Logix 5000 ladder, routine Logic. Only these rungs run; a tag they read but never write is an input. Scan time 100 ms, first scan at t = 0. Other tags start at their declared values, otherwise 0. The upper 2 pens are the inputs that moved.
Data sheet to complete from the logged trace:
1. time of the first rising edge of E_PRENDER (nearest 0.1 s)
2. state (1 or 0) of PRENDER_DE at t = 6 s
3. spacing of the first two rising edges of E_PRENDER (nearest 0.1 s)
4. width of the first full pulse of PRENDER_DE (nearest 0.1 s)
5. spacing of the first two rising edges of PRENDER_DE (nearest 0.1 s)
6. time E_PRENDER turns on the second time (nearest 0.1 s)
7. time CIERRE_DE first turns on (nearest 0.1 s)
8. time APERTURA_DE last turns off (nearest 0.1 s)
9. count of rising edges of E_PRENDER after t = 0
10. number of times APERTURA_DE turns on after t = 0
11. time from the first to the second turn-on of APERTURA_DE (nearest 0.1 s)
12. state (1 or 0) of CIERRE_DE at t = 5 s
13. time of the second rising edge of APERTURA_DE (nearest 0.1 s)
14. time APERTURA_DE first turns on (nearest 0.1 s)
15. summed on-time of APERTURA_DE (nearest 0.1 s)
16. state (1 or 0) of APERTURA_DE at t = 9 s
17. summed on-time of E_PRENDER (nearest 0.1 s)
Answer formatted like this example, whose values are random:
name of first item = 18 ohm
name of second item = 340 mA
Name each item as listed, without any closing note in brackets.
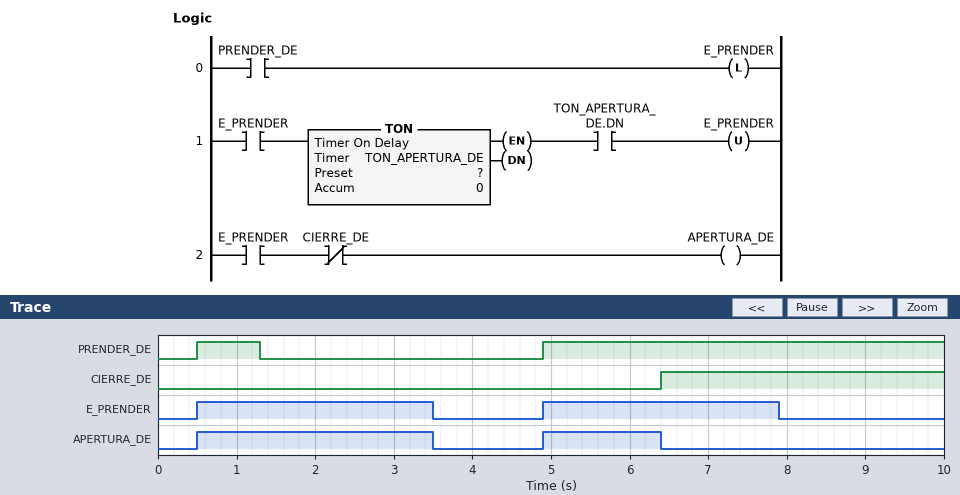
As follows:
time of the first rising edge of E_PRENDER = 0.5 s
state (1 or 0) of PRENDER_DE at t = 6 s = 1
spacing of the first two rising edges of E_PRENDER = 4.4 s
width of the first full pulse of PRENDER_DE = 0.8 s
spacing of the first two rising edges of PRENDER_DE = 4.4 s
time E_PRENDER turns on the second time = 4.9 s
time CIERRE_DE first turns on = 6.4 s
time APERTURA_DE last turns off = 6.4 s
count of rising edges of E_PRENDER after t = 0 = 2
number of times APERTURA_DE turns on after t = 0 = 2
time from the first to the second turn-on of APERTURA_DE = 4.4 s
state (1 or 0) of CIERRE_DE at t = 5 s = 0
time of the second rising edge of APERTURA_DE = 4.9 s
time APERTURA_DE first turns on = 0.5 s
summed on-time of APERTURA_DE = 4.5 s
state (1 or 0) of APERTURA_DE at t = 9 s = 0
summed on-time of E_PRENDER = 6.0 s
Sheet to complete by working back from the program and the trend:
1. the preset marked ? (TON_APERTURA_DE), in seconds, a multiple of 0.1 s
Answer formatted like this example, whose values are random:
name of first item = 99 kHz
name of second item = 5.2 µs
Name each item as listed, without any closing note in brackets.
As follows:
the preset marked ? (TON_APERTURA_DE), in seconds, a multiple of 0.1 s = 3.0 s
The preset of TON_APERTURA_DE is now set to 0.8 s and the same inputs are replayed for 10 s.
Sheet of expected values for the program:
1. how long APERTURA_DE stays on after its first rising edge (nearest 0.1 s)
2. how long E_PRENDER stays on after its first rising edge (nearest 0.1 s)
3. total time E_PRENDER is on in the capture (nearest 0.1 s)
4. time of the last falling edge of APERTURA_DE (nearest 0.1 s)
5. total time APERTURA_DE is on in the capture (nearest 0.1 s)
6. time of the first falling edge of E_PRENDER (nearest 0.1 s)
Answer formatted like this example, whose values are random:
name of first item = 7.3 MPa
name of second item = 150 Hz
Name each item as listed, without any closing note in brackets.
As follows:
how long APERTURA_DE stays on after its first rising edge = 0.8 s
how long E_PRENDER stays on after its first rising edge = 0.8 s
total time E_PRENDER is on in the capture = 1.6 s
time of the last falling edge of APERTURA_DE = 5.7 s
total time APERTURA_DE is on in the capture = 1.6 s
time of the first falling edge of E_PRENDER = 1.3 s
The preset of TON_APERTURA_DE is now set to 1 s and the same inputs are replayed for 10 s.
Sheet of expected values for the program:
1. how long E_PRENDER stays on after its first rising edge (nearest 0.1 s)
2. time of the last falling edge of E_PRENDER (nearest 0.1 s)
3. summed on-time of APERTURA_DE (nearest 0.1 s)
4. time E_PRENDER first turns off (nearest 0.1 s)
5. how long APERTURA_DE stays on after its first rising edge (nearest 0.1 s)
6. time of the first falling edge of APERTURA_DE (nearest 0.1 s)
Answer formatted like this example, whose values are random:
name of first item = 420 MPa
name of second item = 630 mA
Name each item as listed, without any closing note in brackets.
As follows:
how long E_PRENDER stays on after its first rising edge = 1.0 s
time of the last falling edge of E_PRENDER = 5.9 s
summed on-time of APERTURA_DE = 2.0 s
time E_PRENDER first turns off = 1.5 s
how long APERTURA_DE stays on after its first rising edge = 1.0 s
time of the first falling edge of APERTURA_DE = 1.5 s
